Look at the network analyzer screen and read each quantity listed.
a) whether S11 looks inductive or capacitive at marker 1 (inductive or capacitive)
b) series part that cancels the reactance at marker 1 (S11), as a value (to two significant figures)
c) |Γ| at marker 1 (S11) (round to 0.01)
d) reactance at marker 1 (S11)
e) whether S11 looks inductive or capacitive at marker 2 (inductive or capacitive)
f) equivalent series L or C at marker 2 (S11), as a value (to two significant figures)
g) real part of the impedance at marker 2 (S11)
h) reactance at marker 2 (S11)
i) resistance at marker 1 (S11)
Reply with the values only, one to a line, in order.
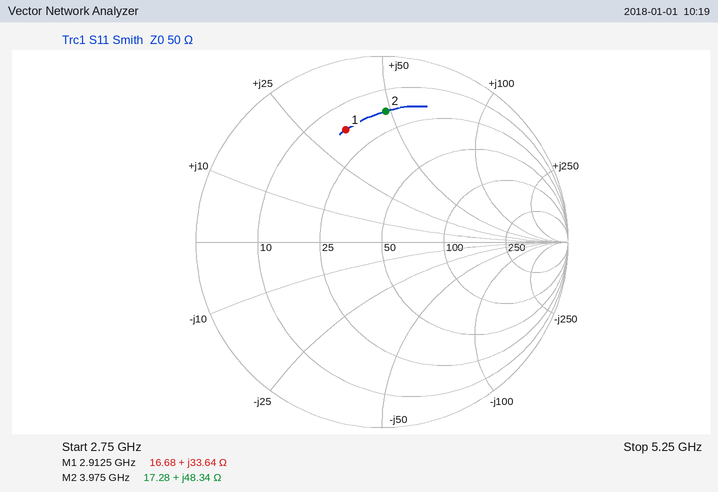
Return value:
inductive
1.6 pF
0.63
+33.64 Ω
inductive
1.9 nH
17.28 Ω
+48.34 Ω
16.68 Ω
